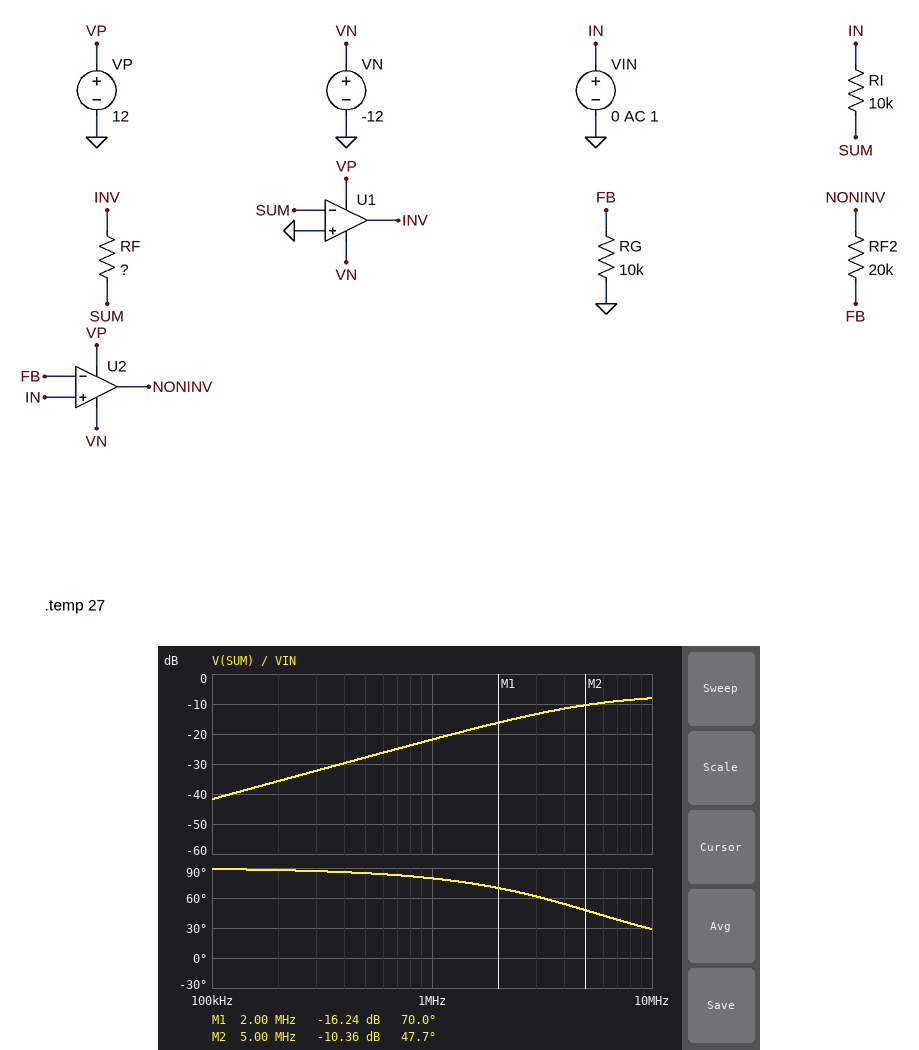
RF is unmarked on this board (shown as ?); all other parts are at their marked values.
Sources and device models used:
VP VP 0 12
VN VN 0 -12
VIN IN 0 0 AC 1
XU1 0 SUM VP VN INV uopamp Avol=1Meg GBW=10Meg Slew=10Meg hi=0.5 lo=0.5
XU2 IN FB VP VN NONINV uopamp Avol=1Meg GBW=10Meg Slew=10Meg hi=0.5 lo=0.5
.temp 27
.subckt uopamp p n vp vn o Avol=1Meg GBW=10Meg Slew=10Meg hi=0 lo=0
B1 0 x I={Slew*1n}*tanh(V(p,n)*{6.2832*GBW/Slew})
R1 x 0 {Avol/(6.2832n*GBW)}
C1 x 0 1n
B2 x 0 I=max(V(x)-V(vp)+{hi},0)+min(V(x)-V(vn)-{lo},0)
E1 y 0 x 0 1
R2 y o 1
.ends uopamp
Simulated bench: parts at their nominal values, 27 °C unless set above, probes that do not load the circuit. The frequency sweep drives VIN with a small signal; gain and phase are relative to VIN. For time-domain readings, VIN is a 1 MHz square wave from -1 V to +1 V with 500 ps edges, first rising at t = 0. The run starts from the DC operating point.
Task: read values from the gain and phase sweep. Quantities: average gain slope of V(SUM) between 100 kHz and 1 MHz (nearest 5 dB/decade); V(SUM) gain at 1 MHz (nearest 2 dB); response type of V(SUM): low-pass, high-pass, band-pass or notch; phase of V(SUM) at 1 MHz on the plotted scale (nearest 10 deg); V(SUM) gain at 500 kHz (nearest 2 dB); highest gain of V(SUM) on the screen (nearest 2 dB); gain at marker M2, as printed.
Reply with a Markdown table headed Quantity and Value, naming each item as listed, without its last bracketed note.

| Quantity | Value |
|---|---|
| average gain slope of V(SUM) between 100 kHz and 1 MHz | 20 dB/decade |
| V(SUM) gain at 1 MHz | -22 dB |
| response type of V(SUM): low-pass, high-pass, band-pass or notch | high-pass |
| phase of V(SUM) at 1 MHz on the plotted scale | 80 deg |
| V(SUM) gain at 500 kHz | -28 dB |
| highest gain of V(SUM) on the screen | -8 dB |
| gain at marker M2, as printed | -10.36 dB |
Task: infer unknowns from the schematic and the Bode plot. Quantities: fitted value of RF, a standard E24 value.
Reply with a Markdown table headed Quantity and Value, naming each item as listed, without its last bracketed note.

| Quantity | Value |
|---|---|
| fitted value of RF, a standard E24 value | 8.2 kΩ |
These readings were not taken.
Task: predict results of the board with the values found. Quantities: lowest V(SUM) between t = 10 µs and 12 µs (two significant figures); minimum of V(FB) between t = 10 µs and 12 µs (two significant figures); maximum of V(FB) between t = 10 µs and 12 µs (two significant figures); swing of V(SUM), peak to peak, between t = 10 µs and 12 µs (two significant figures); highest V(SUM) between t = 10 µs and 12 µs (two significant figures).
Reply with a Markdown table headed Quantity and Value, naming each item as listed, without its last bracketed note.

| Quantity | Value |
|---|---|
| lowest V(SUM) between t = 10 µs and 12 µs | -900 mV |
| minimum of V(FB) between t = 10 µs and 12 µs | -830 mV |
| maximum of V(FB) between t = 10 µs and 12 µs | 820 mV |
| swing of V(SUM), peak to peak, between t = 10 µs and 12 µs | 1.8 V |
| highest V(SUM) between t = 10 µs and 12 µs | 900 mV |
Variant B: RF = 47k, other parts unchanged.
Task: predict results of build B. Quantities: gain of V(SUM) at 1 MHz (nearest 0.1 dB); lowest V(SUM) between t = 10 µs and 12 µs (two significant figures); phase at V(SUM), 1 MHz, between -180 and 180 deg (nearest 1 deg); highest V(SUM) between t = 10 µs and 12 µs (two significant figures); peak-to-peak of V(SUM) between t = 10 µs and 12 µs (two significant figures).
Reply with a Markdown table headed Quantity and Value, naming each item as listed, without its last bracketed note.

| Quantity | Value |
|---|---|
| gain of V(SUM) at 1 MHz | -7.8 dB |
| lowest V(SUM) between t = 10 µs and 12 µs | -1.1 V |
| phase at V(SUM), 1 MHz, between -180 and 180 deg | 60 deg |
| highest V(SUM) between t = 10 µs and 12 µs | 1.4 V |
| peak-to-peak of V(SUM) between t = 10 µs and 12 µs | 2.5 V |
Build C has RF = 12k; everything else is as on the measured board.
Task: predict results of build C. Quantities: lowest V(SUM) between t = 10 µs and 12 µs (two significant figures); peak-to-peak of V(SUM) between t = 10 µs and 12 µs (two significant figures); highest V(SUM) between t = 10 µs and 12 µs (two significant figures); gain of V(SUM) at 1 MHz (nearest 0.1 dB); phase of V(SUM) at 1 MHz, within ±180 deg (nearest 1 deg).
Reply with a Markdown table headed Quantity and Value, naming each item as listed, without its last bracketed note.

| Quantity | Value |
|---|---|
| lowest V(SUM) between t = 10 µs and 12 µs | -1.1 V |
| peak-to-peak of V(SUM) between t = 10 µs and 12 µs | 2.2 V |
| highest V(SUM) between t = 10 µs and 12 µs | 1.1 V |
| gain of V(SUM) at 1 MHz | -18.6 dB |
| phase of V(SUM) at 1 MHz, within ±180 deg | 78 deg |
